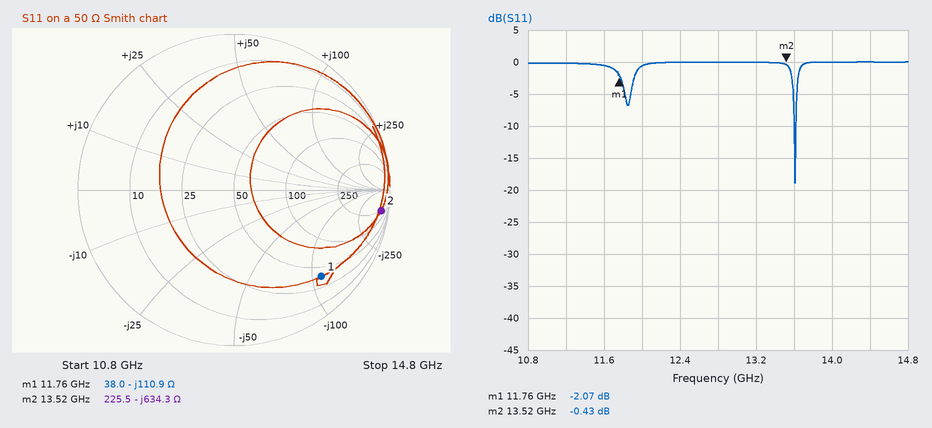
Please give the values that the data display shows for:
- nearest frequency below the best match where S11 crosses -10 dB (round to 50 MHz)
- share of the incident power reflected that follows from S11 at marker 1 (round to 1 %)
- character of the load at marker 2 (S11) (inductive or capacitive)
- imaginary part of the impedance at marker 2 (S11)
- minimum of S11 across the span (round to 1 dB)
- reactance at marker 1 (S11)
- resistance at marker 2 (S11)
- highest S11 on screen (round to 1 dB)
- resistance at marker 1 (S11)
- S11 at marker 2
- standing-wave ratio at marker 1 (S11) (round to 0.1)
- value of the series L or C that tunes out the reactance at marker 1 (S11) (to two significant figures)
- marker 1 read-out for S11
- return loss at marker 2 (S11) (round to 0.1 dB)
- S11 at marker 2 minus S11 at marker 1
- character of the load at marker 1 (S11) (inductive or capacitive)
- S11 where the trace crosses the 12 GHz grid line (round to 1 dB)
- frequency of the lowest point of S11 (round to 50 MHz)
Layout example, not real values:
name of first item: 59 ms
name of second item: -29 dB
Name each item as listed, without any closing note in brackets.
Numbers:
nearest frequency below the best match where S11 crosses -10 dB: 13.60 GHz
share of the incident power reflected that follows from S11 at marker 1: 62 %
character of the load at marker 2 (S11): capacitive
imaginary part of the impedance at marker 2: -634.3 Ω
minimum of S11 across the span: -19 dB
reactance at marker 1: -110.9 Ω
resistance at marker 2: 225.5 Ω
highest S11 on screen: 0 dB
resistance at marker 1: 38.0 Ω
S11 at marker 2: -0.43 dB
standing-wave ratio at marker 1 (S11): 8.4
value of the series L or C that tunes out the reactance at marker 1 (S11): 1.5 nH
marker 1 read-out for S11: -2.07 dB
return loss at marker 2 (S11): 0.4 dB
S11 at marker 2 minus S11 at marker 1: 1.64 dB
character of the load at marker 1 (S11): capacitive
S11 where the trace crosses the 12 GHz grid line: -1 dB
frequency of the lowest point of S11: 13.60 GHz
